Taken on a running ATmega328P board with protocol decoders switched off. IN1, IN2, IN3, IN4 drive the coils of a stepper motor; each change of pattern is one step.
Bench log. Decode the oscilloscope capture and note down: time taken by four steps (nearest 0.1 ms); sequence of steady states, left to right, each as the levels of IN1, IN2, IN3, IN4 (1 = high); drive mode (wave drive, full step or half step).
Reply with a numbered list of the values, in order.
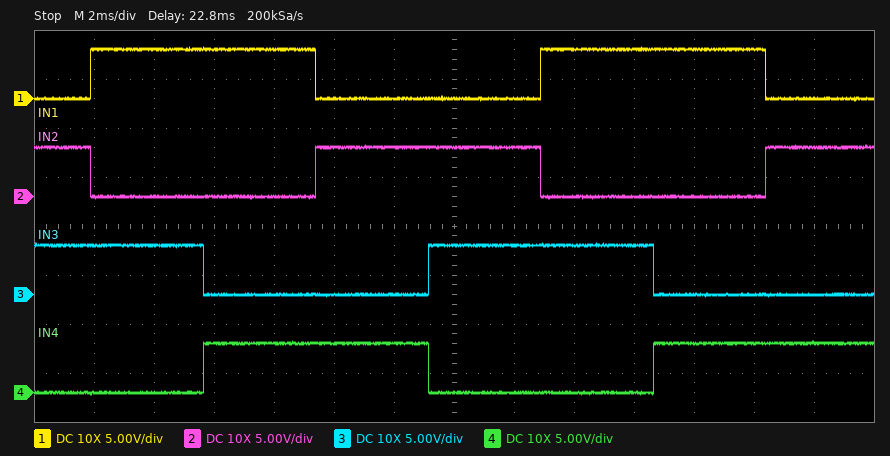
1. 15.0 ms
2. 0110 1010 1001 0101 0110 1010 1001 0101
3. full step
